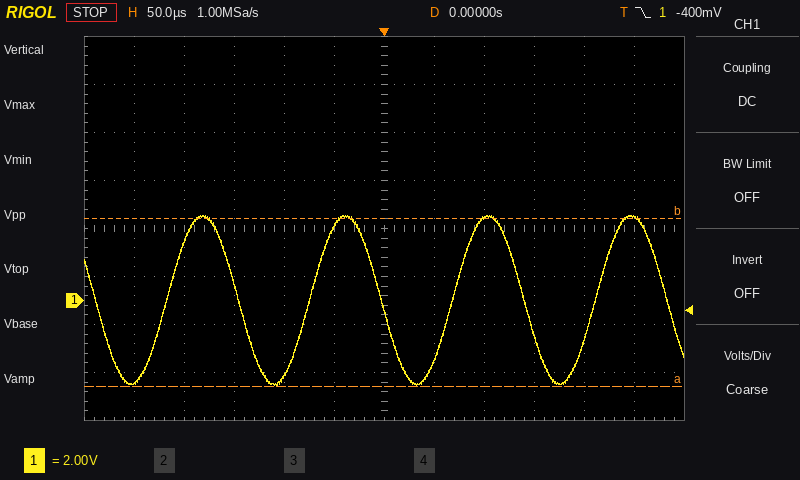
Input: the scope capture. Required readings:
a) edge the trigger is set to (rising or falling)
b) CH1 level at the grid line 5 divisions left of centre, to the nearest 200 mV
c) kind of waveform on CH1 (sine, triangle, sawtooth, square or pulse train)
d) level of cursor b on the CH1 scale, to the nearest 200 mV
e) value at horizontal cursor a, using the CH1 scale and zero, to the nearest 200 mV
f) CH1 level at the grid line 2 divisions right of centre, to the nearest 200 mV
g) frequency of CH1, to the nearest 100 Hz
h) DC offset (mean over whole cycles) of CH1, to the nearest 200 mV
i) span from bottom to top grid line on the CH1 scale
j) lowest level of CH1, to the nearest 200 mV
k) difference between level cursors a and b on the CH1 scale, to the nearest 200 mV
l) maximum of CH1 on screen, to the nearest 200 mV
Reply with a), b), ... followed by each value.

a) falling
b) -3.4 V
c) sine
d) 3.4 V
e) -3.6 V
f) 3.4 V
g) 7.0 kHz
h) 0.0 V
i) 16 V
j) -3.6 V
k) 7.0 V
l) 3.6 V
